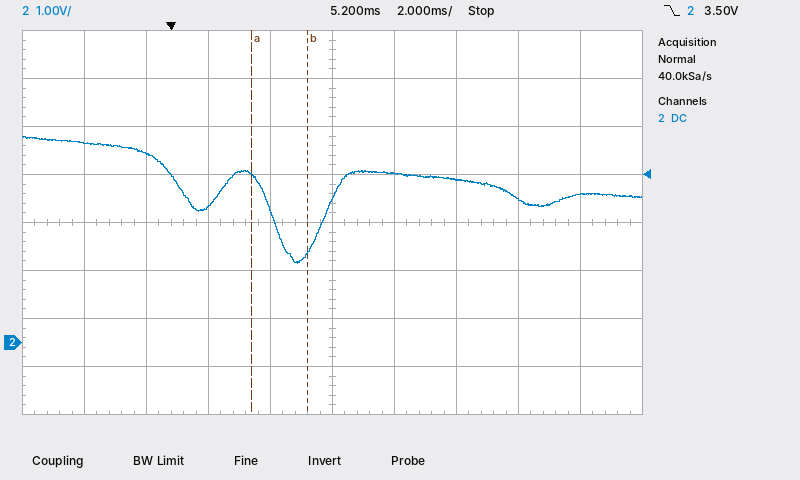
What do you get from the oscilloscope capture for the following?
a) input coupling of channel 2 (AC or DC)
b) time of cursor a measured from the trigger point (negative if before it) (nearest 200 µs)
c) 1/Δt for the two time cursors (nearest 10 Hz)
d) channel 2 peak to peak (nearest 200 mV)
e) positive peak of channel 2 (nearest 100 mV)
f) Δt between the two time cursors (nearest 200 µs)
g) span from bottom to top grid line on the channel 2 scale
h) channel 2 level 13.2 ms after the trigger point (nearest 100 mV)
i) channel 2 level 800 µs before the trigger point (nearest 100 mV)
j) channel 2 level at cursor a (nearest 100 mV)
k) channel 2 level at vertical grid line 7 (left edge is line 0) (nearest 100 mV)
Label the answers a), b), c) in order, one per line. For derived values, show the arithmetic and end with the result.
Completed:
a) DC
b) +2.6 ms
c) 1 / 1.8 ms ≈ 560 Hz
d) 2.6 V
e) 4.3 V
f) 1.8 ms
g) 8 V
h) 3.1 V
i) 3.9 V
j) 3.5 V
k) 3.4 V
